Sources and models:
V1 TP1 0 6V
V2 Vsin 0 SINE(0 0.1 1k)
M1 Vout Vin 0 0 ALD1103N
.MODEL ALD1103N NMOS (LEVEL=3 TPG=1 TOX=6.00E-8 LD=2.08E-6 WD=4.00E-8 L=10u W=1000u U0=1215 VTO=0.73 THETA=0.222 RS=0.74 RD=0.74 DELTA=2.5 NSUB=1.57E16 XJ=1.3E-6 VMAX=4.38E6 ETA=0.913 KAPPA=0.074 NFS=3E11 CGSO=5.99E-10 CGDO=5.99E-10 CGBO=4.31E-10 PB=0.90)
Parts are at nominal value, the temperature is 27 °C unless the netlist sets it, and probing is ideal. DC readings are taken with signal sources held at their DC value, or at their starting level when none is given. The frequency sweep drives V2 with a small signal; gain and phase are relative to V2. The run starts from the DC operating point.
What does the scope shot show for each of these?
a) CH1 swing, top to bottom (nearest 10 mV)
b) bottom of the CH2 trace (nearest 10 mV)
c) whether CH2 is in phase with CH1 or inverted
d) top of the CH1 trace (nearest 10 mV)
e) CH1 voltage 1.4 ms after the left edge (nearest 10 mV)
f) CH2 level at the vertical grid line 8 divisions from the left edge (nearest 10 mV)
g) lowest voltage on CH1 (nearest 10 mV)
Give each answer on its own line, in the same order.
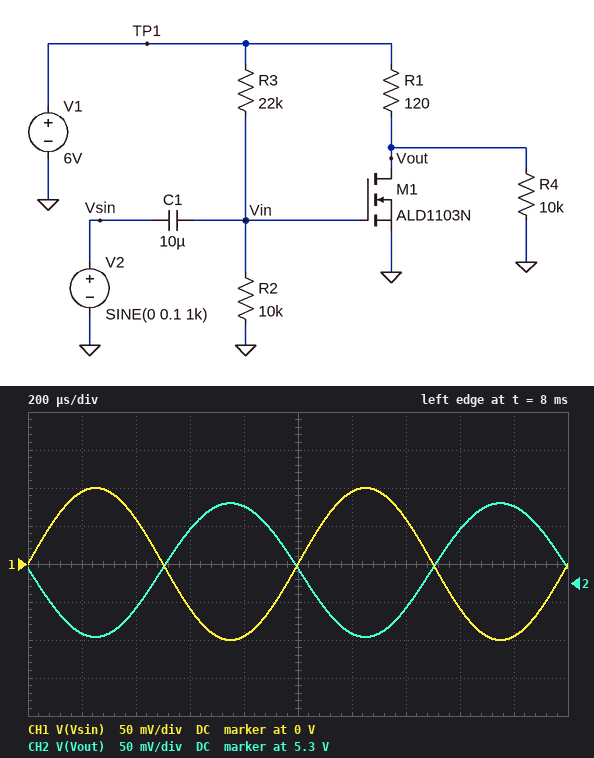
200 mV
5.23 V
inverted
100 mV
60 mV
5.37 V
-100 mV
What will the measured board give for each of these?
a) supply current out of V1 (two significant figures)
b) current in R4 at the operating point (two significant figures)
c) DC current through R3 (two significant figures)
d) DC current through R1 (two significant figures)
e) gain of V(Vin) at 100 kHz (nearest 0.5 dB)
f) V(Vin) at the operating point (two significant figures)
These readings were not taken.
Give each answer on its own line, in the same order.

5.9 mA
530 µA
190 µA
5.7 mA
0 dB
1.9 V
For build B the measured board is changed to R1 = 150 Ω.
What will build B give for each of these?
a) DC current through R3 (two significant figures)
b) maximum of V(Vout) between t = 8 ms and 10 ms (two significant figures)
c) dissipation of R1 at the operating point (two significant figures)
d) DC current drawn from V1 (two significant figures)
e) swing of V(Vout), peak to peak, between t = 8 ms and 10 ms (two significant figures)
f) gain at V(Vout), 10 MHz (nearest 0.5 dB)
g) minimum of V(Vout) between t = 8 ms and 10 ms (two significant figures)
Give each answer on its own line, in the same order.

190 µA
5.3 V
4.8 mW
5.8 mA
220 mV
1.0 dB
5.0 V
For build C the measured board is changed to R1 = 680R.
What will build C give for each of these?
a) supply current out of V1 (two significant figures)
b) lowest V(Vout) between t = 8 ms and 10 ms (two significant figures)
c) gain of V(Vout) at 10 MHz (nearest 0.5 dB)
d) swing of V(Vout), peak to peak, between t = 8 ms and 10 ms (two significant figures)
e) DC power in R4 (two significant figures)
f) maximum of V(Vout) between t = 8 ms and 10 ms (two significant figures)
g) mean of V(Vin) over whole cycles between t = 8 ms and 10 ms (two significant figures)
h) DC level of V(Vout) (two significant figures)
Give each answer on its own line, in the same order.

5.4 mA
2.0 V
13.0 dB
910 mV
590 µW
2.9 V
1.9 V
2.4 V
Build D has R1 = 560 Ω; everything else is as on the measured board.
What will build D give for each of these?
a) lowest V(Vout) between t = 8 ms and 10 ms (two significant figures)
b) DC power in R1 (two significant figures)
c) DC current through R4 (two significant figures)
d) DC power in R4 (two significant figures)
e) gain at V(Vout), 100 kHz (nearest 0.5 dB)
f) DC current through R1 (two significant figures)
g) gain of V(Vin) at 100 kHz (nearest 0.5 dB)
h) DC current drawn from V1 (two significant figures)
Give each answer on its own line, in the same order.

2.6 V
16 mW
300 µA
910 µW
11.5 dB
5.3 mA
0 dB
5.5 mA
